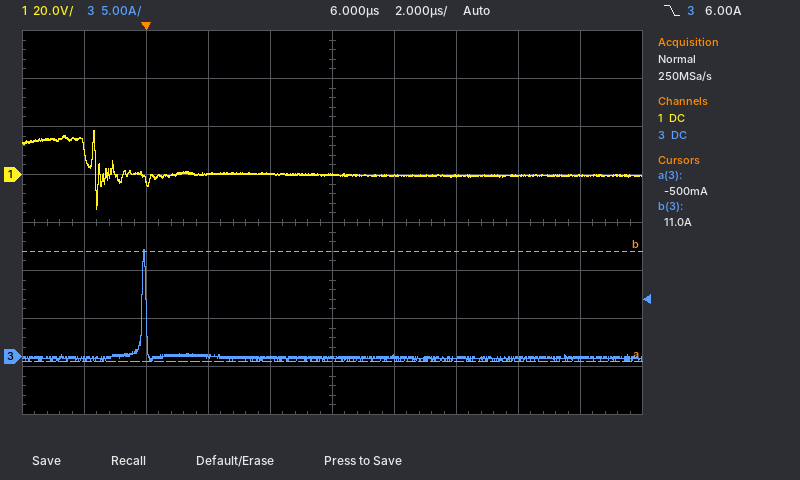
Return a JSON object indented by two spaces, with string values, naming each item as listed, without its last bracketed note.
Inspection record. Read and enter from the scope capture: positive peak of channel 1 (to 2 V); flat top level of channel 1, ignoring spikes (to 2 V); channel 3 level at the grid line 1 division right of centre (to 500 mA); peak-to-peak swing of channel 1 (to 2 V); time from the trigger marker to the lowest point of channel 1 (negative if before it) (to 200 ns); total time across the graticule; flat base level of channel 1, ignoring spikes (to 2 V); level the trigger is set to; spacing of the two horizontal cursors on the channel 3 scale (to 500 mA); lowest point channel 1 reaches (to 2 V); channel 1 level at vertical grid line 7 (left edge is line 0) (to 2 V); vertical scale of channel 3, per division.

{
  "positive peak of channel 1": "18 V",
  "flat top level of channel 1, ignoring spikes": "14 V",
  "channel 3 level at the grid line 1 division right of centre": "0.0 A",
  "peak-to-peak swing of channel 1": "32 V",
  "time from the trigger marker to the lowest point of channel 1 (negative if before it)": "-1.6 µs",
  "total time across the graticule": "20 µs",
  "flat base level of channel 1, ignoring spikes": "0 V",
  "level the trigger is set to": "6.00 A",
  "spacing of the two horizontal cursors on the channel 3 scale": "11.5 A",
  "lowest point channel 1 reaches": "-14 V",
  "channel 1 level at vertical grid line 7 (left edge is line 0)": "0 V",
  "vertical scale of channel 3, per division": "5 A"
}
